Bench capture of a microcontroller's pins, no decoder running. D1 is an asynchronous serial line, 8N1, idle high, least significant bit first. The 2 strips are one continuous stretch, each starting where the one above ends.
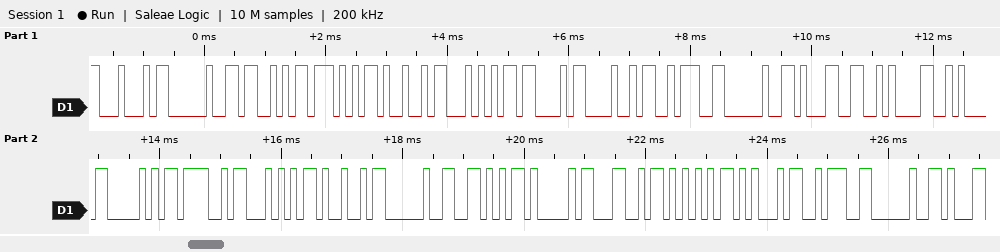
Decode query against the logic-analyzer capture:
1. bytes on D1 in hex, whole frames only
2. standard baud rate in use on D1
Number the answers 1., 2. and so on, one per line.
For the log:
1. 44 20 53 57 49 54 43 48 3A 20 31 0A 0A 50 4F 54 49 20 56 41 4C 55 45 3A 20
2. 9600 baud
